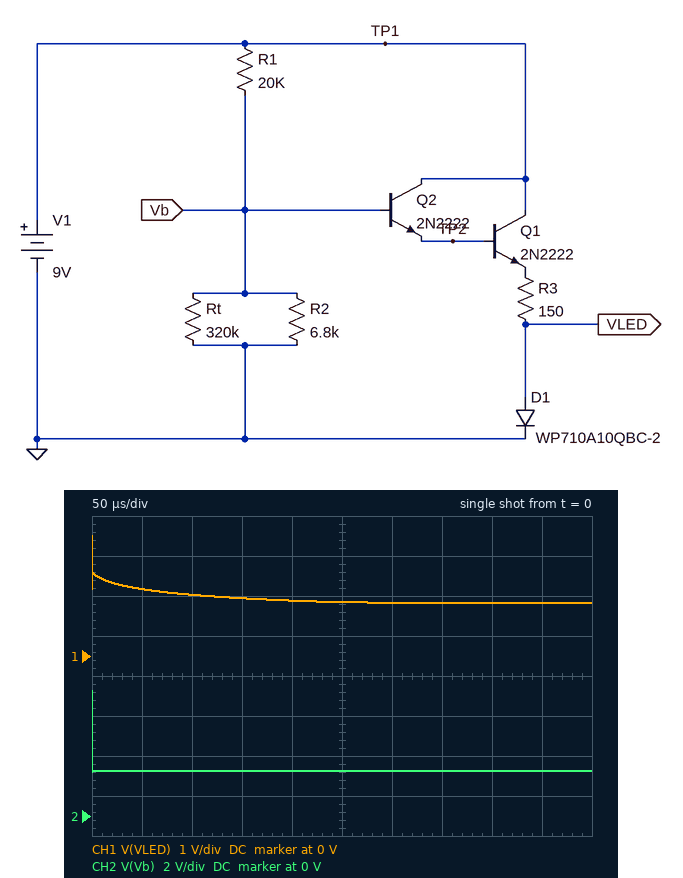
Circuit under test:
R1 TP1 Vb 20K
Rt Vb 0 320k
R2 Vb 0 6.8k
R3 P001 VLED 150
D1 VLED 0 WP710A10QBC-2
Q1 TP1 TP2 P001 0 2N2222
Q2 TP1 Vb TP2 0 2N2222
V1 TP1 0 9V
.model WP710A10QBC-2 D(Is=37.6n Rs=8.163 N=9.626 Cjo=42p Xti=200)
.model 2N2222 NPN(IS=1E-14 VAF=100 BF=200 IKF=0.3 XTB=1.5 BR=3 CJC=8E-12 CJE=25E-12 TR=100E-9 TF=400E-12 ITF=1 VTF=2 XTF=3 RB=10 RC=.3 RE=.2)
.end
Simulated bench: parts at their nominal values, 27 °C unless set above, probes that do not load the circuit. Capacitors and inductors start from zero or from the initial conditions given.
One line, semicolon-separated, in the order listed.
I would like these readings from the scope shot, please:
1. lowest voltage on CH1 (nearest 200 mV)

1.4 V
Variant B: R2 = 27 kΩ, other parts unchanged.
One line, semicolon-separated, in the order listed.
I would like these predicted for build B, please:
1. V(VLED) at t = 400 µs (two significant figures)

3.0 V
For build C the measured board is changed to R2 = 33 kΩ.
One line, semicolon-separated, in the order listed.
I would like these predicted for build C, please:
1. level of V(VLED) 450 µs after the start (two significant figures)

3.1 V
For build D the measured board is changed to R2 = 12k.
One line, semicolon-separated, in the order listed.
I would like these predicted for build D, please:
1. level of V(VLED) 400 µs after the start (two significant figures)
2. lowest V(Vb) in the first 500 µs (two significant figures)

2.2 V; 3.3 V
